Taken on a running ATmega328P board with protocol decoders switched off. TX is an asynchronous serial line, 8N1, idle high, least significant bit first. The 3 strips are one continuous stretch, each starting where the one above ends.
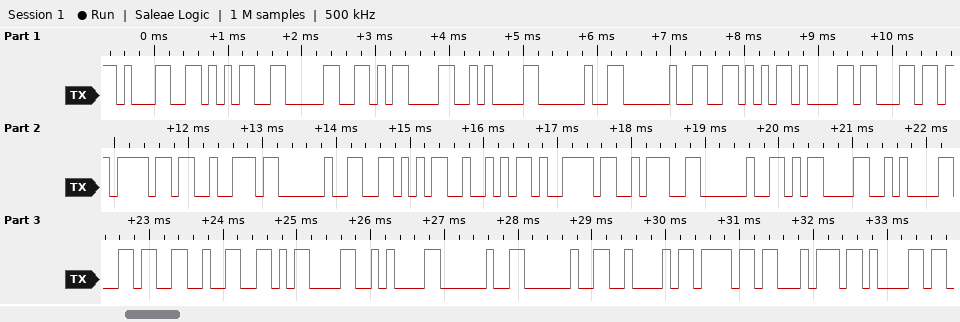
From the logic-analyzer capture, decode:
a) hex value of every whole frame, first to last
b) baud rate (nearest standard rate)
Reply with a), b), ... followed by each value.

a) 31 35 30 0D 0A 20 20 56 61 6C 6F 72 20 56 52 79 3A 20 0D 0A 36 32 0D 0A 20 20 42 6F 74 61
b) 9600 baud
